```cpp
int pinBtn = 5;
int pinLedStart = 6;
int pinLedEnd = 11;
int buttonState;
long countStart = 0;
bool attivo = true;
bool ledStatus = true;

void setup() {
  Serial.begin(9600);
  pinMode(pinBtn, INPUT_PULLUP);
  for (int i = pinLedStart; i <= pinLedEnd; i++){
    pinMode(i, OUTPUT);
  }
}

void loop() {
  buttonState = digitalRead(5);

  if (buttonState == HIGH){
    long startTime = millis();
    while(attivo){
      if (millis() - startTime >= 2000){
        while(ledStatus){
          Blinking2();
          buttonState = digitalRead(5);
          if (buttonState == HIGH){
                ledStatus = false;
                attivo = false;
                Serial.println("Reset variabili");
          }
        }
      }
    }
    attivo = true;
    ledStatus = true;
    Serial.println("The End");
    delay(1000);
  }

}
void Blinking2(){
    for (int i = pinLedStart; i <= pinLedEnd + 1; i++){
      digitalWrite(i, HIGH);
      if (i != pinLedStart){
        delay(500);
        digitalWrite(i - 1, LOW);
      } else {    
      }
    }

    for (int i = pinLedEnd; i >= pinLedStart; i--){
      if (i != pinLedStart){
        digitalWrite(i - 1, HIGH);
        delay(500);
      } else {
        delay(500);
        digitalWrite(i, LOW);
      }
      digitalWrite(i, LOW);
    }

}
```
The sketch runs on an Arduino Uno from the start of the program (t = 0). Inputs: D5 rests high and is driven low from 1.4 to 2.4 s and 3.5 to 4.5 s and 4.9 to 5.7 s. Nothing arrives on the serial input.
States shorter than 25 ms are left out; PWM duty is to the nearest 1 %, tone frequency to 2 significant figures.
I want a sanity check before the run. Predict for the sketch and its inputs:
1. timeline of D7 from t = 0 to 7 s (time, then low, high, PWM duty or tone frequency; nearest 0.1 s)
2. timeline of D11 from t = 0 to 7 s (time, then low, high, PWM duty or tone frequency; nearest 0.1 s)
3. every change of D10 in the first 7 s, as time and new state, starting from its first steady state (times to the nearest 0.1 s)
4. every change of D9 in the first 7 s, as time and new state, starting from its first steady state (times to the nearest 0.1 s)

0 s low; 2 s high; 3 s low; 6.5 s high
0 s low; 4 s high; 5 s low
0 s low; 3.5 s high; 4.5 s low; 5 s high; 6 s low
0 s low; 3 s high; 4 s low; 5.5 s high; 6.5 s low
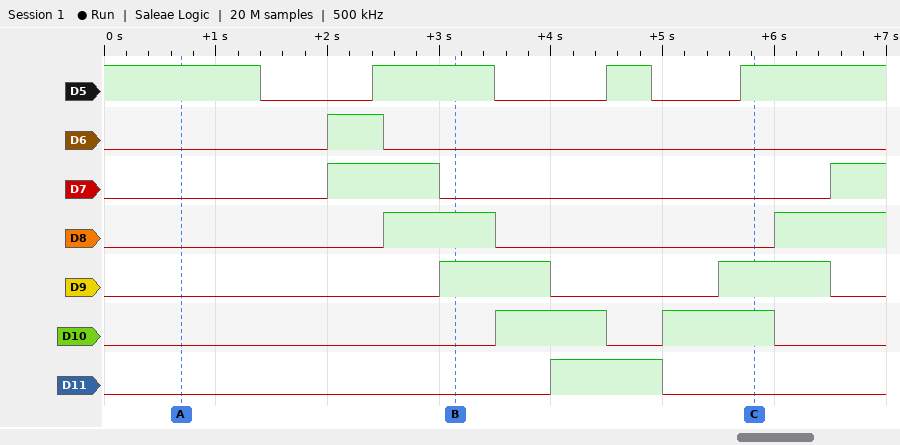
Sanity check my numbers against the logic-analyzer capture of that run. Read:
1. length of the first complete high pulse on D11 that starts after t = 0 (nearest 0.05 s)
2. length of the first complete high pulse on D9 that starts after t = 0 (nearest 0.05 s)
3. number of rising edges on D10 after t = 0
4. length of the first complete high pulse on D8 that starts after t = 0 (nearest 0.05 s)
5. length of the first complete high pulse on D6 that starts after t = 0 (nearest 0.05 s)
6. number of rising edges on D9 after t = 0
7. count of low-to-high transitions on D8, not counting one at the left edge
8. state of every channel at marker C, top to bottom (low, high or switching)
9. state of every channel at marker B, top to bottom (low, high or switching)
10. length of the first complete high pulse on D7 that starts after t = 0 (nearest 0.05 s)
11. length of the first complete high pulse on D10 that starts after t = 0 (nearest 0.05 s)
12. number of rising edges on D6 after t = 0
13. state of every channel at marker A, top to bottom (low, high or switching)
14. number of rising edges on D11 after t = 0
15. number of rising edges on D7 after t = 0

1.00 s
1.00 s
2
1.00 s
0.50 s
2
2
D5 high, D6 low, D7 low, D8 low, D9 high, D10 high, D11 low
D5 high, D6 low, D7 low, D8 high, D9 high, D10 low, D11 low
1.00 s
1.00 s
1
D5 high, D6 low, D7 low, D8 low, D9 low, D10 low, D11 low
1
2
